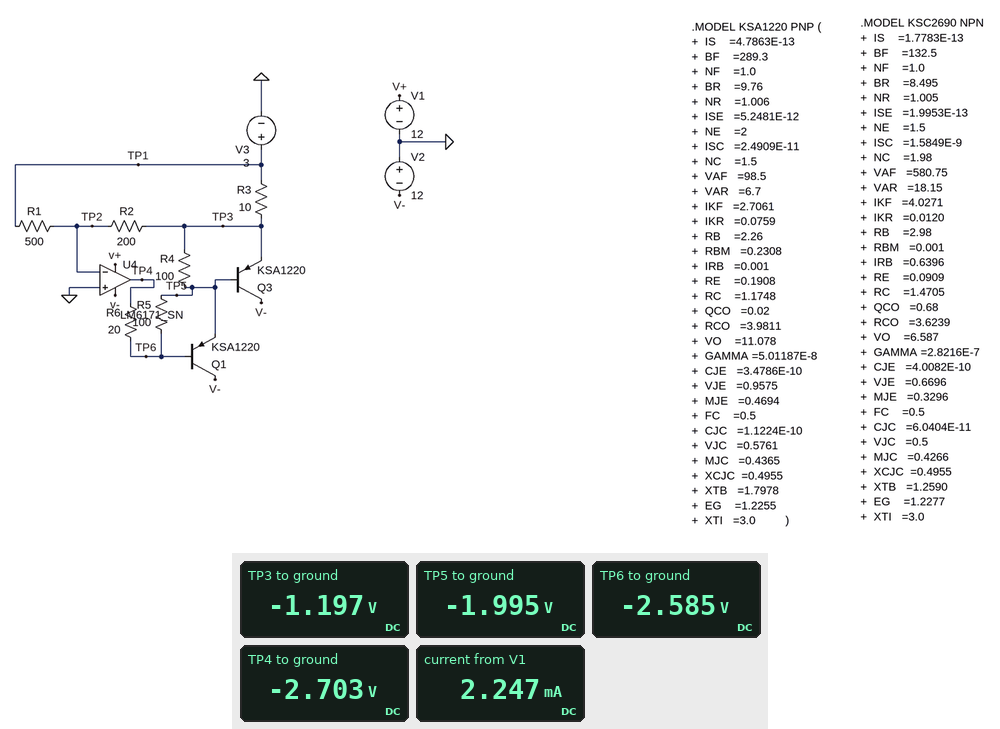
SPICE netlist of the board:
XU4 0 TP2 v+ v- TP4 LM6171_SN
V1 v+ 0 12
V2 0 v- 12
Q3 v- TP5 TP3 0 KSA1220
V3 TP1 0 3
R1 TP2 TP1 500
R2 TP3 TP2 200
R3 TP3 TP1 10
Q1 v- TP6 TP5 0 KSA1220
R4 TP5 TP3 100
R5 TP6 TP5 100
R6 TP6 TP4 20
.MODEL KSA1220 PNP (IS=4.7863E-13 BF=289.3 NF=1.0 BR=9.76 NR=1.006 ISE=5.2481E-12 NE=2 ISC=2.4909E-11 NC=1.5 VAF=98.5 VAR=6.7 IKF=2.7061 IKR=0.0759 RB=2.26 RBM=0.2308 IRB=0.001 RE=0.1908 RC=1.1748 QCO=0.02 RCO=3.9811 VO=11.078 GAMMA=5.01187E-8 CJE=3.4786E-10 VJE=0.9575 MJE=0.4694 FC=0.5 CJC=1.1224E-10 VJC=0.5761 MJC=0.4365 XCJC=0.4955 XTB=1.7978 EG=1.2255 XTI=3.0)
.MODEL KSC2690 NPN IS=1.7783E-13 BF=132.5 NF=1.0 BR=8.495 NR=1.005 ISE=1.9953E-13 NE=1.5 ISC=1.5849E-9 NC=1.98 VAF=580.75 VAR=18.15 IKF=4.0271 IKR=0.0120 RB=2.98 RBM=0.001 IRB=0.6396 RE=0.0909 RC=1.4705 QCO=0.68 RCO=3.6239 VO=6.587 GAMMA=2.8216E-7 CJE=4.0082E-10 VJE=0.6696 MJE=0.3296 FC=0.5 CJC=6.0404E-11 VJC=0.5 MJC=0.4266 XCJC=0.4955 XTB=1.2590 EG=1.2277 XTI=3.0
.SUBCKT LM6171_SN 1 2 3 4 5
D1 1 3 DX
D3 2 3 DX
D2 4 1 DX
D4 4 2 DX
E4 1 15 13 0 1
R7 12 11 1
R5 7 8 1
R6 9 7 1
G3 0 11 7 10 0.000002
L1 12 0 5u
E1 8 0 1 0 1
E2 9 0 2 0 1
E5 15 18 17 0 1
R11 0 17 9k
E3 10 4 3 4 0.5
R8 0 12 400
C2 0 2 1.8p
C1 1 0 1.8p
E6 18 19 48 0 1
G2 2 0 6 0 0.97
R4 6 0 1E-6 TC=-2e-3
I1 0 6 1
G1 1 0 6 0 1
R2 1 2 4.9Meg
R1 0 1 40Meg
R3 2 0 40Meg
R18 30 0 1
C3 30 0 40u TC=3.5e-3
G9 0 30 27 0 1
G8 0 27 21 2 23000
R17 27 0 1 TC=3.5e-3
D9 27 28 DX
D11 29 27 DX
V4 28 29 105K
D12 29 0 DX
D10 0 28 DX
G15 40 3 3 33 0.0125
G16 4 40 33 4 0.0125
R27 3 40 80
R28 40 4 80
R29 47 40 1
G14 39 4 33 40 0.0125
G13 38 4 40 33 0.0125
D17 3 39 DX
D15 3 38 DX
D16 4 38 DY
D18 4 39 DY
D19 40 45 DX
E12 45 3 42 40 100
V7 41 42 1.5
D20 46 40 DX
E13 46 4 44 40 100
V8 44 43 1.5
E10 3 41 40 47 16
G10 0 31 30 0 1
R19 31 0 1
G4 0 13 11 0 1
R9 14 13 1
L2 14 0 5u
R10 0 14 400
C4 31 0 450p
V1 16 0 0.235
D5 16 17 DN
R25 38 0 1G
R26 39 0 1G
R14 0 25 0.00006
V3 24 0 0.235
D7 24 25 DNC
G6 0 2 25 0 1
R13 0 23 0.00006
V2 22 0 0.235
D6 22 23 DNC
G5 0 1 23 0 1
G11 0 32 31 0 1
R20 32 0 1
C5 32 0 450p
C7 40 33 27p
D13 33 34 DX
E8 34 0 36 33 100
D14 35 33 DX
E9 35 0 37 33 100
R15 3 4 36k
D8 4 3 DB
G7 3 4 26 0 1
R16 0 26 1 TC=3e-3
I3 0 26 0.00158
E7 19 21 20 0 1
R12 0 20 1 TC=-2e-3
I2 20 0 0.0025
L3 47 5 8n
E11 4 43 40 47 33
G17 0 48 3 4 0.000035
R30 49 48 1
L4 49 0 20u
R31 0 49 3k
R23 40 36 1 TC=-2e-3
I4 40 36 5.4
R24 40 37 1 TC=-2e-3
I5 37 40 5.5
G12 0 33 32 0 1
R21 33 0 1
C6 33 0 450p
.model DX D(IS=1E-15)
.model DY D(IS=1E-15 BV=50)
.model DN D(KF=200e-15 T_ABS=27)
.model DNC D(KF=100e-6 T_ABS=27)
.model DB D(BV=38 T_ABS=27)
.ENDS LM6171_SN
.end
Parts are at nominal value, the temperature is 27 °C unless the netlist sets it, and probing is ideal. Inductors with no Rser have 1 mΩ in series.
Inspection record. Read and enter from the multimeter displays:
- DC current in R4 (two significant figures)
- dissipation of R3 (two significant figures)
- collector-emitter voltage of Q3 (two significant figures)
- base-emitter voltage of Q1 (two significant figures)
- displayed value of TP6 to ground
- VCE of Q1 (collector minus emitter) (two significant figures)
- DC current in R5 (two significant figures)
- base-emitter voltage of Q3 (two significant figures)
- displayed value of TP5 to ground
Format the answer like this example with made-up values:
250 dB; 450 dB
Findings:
8.0 mA; 1.8 W; -11 V; -590 mV; -2.585 V; -10 V; 5.9 mA; -800 mV; -1.995 V
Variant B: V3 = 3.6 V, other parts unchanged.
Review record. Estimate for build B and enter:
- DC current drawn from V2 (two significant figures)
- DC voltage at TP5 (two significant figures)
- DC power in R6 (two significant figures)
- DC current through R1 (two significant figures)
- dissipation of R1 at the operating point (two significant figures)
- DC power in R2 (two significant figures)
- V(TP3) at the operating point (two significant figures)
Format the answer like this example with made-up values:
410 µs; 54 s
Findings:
510 mA; -2.3 V; 710 µW; 7.2 mA; 26 mW; 10 mW; -1.4 V
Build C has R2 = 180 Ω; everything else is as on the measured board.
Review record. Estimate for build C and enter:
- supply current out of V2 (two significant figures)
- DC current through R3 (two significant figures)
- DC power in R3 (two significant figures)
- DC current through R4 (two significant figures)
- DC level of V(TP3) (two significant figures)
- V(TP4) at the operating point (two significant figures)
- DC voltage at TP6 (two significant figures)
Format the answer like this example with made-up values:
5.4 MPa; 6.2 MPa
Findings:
420 mA; 410 mA; 1.7 W; 7.9 mA; -1.1 V; -2.6 V; -2.5 V
